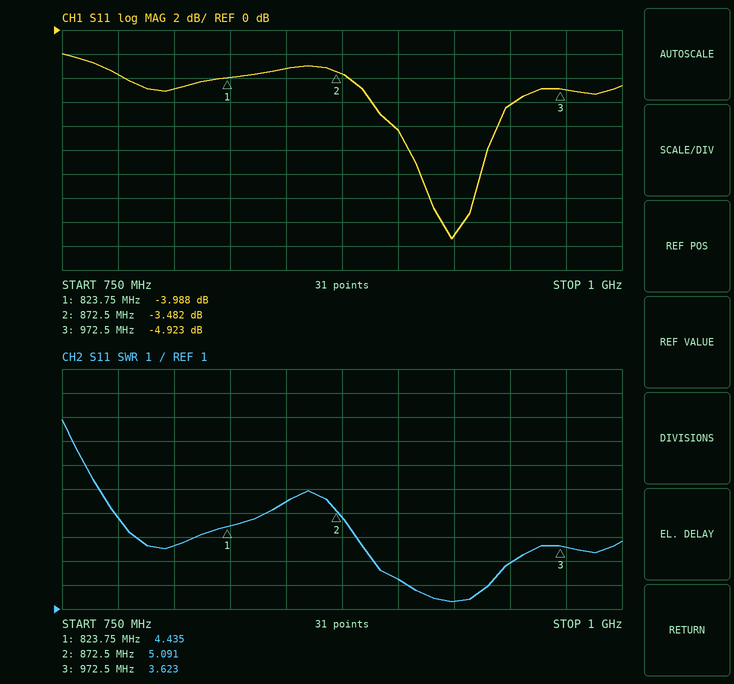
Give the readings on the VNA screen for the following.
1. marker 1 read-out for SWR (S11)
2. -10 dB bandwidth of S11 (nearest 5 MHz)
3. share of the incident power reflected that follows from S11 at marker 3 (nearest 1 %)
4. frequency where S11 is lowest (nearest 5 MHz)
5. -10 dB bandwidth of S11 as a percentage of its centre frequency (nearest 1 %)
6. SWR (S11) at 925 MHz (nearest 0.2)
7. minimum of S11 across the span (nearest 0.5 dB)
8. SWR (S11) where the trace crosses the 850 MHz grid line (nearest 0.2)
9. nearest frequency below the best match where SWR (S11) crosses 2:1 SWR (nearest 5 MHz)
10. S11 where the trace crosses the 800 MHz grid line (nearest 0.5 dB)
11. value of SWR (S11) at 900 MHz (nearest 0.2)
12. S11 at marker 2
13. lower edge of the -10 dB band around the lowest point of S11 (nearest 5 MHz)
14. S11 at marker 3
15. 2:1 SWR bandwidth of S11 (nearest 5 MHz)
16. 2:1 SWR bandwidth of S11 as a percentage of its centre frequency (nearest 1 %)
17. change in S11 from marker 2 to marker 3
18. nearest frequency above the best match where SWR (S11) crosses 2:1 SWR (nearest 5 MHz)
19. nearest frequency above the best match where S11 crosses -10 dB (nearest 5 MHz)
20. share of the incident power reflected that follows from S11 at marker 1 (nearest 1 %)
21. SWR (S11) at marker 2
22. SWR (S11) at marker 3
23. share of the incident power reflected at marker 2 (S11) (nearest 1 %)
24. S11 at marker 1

4.435
35 MHz
32 %
925 MHz
4 %
1.4
-17.5 dB
5.4
905 MHz
-5.0 dB
2.2
-3.482 dB
905 MHz
-4.923 dB
35 MHz
4 %
-1.441 dB
940 MHz
940 MHz
40 %
5.091
3.623
45 %
-3.988 dB
